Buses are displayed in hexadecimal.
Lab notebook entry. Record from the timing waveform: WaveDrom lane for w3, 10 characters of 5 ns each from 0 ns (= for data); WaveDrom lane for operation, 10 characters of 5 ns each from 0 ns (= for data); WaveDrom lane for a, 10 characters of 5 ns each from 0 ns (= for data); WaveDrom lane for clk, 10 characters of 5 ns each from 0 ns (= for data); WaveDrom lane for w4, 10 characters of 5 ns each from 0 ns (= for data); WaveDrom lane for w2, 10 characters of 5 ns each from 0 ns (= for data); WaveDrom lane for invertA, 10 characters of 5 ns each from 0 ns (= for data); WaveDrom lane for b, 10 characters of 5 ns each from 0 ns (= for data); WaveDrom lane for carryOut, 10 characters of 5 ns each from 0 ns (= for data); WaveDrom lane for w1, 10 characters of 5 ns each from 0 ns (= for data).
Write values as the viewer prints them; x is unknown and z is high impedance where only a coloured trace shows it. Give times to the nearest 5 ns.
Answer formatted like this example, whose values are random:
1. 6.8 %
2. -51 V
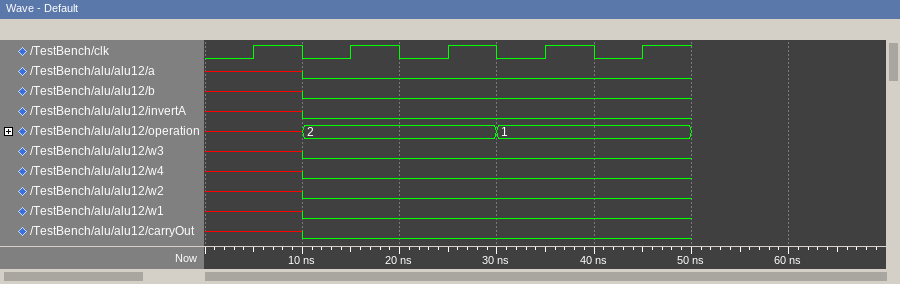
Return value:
1. {name: 'w3', wave: 'x.0.......'}
2. {name: 'operation', wave: 'x.=...=...', data: '2 1'}
3. {name: 'a', wave: 'x.0.......'}
4. {name: 'clk', wave: '0101010101'}
5. {name: 'w4', wave: 'x.0.......'}
6. {name: 'w2', wave: 'x.0.......'}
7. {name: 'invertA', wave: 'x.0.......'}
8. {name: 'b', wave: 'x.0.......'}
9. {name: 'carryOut', wave: 'x.0.......'}
10. {name: 'w1', wave: 'x.0.......'}
